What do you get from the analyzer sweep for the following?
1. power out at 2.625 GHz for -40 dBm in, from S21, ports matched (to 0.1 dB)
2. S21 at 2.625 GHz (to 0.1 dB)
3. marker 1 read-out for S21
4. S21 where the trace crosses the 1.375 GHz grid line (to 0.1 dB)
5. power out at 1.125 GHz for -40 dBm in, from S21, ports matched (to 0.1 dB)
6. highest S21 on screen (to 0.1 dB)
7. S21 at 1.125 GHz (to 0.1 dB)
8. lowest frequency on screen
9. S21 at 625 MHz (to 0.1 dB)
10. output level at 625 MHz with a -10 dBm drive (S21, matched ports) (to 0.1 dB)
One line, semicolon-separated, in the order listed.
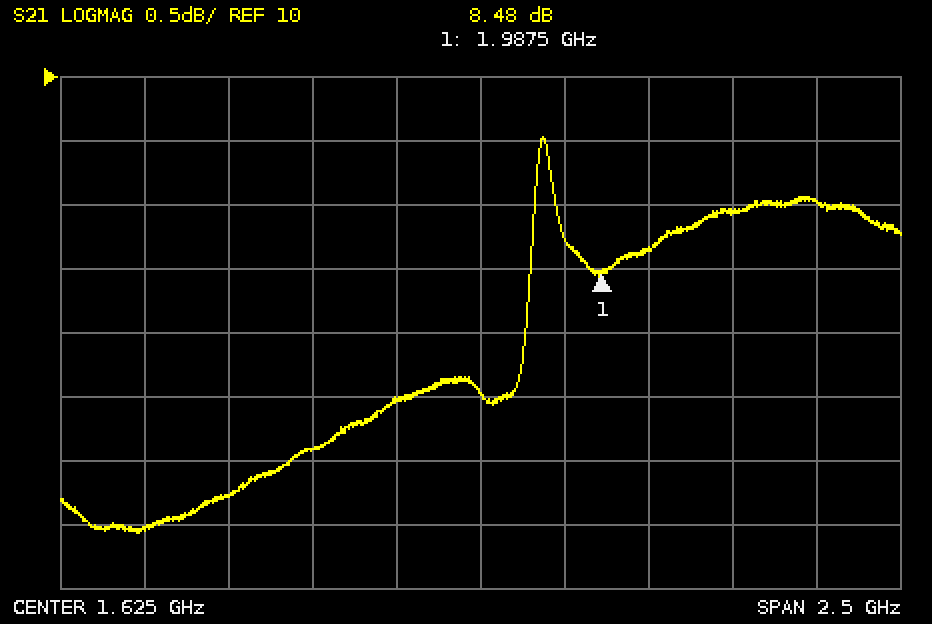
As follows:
-31.0 dBm; 9.0 dB; 8.48 dB; 7.5 dB; -32.9 dBm; 9.5 dB; 7.1 dB; 375 MHz; 6.5 dB; -3.5 dBm
